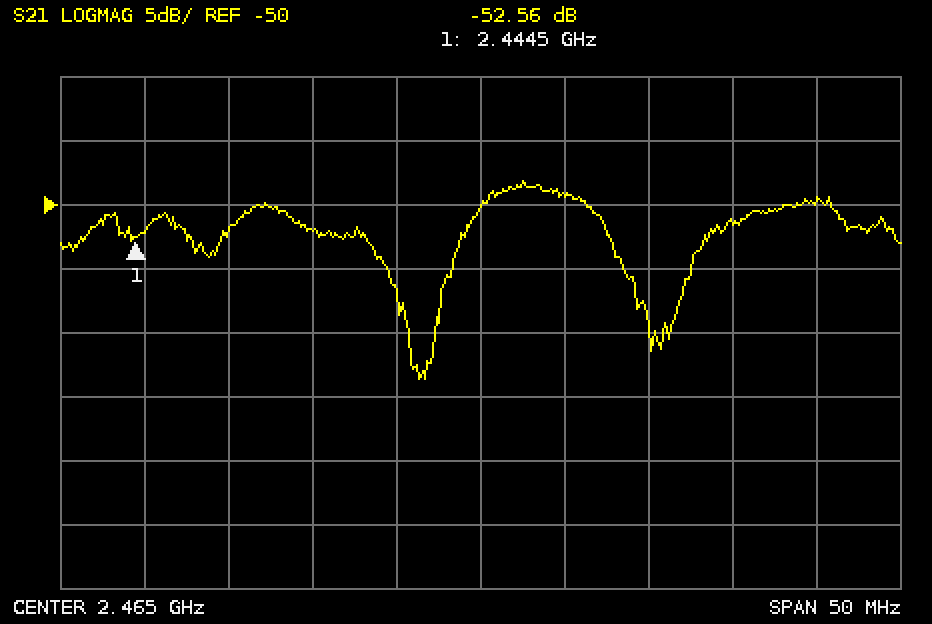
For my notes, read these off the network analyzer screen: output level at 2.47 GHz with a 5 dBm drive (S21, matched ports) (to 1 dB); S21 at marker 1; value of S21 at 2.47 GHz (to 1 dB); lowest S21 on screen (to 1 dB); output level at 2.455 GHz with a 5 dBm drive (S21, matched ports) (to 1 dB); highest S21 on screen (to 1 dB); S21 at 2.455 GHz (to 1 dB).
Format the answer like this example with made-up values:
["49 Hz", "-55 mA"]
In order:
["-44 dBm", "-52.56 dB", "-49 dB", "-64 dB", "-47 dBm", "-48 dB", "-52 dB"]
